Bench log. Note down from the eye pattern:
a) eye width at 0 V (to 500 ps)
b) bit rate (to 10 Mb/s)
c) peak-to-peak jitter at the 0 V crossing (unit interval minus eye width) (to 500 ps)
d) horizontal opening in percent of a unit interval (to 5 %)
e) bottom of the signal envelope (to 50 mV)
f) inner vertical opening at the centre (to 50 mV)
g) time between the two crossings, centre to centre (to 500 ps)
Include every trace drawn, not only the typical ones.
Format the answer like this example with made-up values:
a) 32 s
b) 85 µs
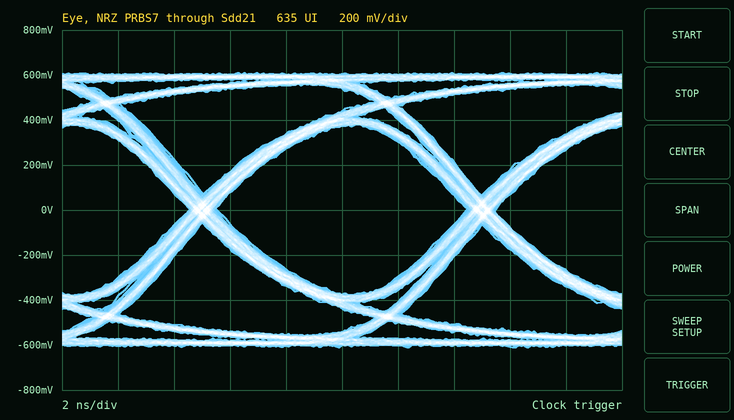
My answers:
a) 9.0 ns
b) 100 Mb/s
c) 1.0 ns
d) 90 %
e) -600 mV
f) 750 mV
g) 10.0 ns
